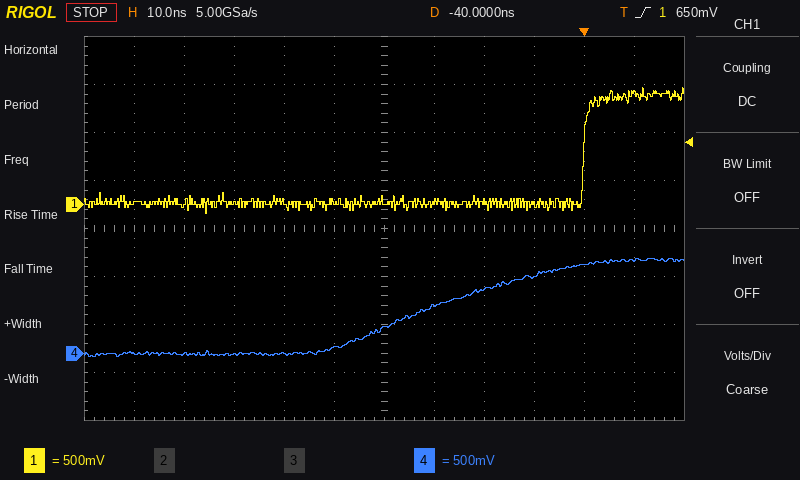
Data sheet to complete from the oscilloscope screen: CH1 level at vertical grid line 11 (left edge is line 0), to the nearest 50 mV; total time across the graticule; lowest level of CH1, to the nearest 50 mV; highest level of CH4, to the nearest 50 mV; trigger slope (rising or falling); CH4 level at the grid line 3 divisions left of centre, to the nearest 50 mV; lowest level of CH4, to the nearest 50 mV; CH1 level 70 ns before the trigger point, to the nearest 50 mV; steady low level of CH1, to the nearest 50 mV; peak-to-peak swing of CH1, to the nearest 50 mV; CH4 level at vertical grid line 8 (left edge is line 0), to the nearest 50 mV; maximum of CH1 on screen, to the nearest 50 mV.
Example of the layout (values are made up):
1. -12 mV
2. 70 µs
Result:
1. 1.15 V
2. 120 ns
3. -100 mV
4. 1.00 V
5. rising
6. 0 mV
7. -50 mV
8. 0 mV
9. 0 mV
10. 1.30 V
11. 650 mV
12. 1.20 V
